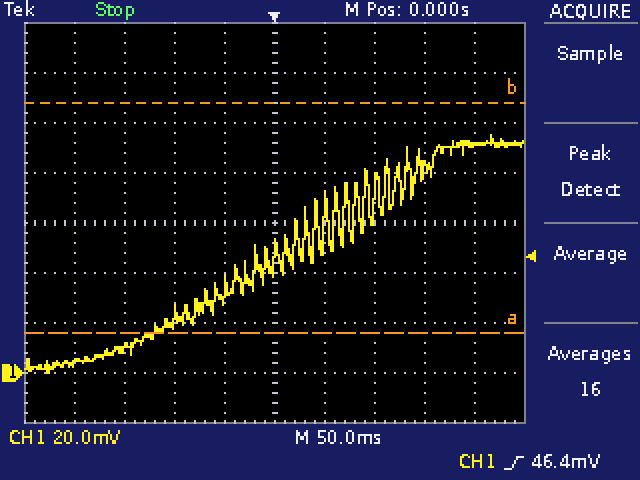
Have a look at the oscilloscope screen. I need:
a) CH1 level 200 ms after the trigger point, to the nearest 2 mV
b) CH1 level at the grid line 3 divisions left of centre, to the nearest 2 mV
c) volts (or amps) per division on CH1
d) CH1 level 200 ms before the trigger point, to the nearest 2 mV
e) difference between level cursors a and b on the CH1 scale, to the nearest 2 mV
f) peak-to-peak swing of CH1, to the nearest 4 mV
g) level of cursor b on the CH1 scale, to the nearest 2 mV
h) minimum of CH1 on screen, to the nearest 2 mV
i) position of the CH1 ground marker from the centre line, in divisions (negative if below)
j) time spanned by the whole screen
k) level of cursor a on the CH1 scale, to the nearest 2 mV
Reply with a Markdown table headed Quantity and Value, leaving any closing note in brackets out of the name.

| Quantity | Value |
|---|---|
| CH1 level 200 ms after the trigger point, to the nearest 2 mV | 92 mV |
| CH1 level at the grid line 3 divisions left of centre, to the nearest 2 mV | 10 mV |
| volts (or amps) per division on CH1 | 20 mV |
| CH1 level 200 ms before the trigger point, to the nearest 2 mV | 4 mV |
| difference between level cursors a and b on the CH1 scale, to the nearest 2 mV | 92 mV |
| peak-to-peak swing of CH1, to the nearest 4 mV | 96 mV |
| level of cursor b on the CH1 scale, to the nearest 2 mV | 108 mV |
| minimum of CH1 on screen, to the nearest 2 mV | 0 mV |
| position of the CH1 ground marker from the centre line, in divisions | -3.0 div |
| time spanned by the whole screen | 500 ms |
| level of cursor a on the CH1 scale, to the nearest 2 mV | 16 mV |
